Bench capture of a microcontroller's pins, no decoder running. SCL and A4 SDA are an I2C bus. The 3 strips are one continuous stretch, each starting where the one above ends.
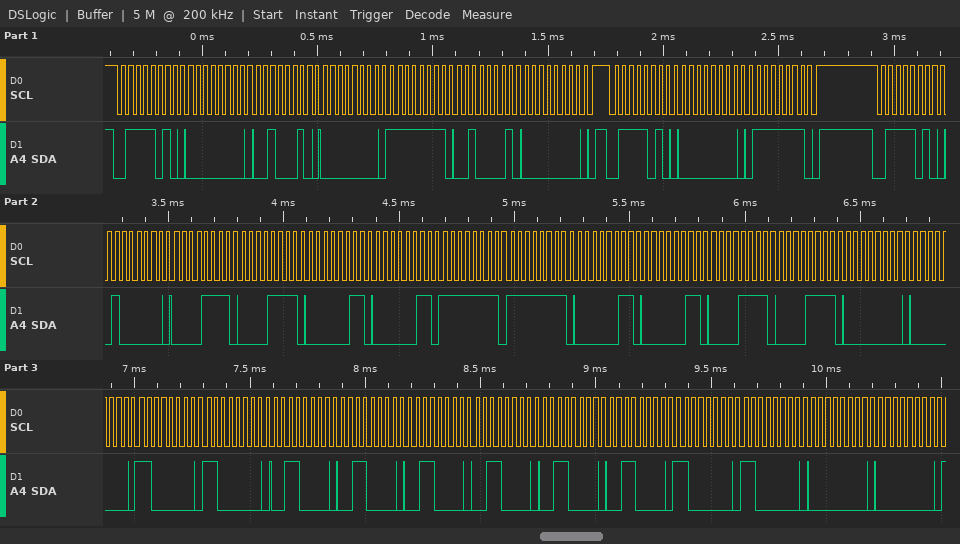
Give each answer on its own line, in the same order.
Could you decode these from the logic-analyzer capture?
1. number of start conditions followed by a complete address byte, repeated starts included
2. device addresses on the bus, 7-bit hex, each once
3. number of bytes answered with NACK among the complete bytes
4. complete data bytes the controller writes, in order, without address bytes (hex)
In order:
3
0x3D
0
00 22 00 FF 21 00 00 7F 40 0F 0F 03 03 FF FF 03 03 0F 0F 00 00 C0 C0 30 30 30 30 30 30 C0 C0 00 00
